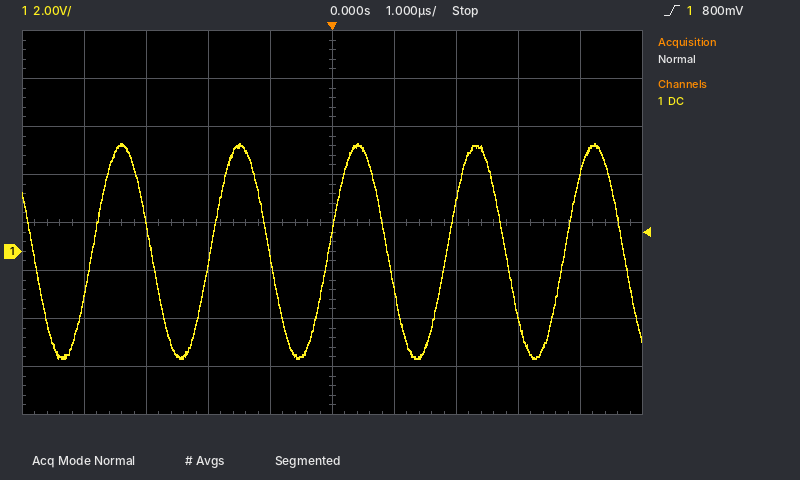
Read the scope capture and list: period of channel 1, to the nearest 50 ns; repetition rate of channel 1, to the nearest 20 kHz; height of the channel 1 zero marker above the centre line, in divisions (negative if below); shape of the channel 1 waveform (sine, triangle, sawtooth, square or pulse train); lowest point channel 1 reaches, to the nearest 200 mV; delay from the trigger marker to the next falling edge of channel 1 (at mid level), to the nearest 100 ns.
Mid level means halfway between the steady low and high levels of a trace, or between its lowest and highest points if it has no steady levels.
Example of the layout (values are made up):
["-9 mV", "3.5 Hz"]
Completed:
["1.90 µs", "520 kHz", "-0.6 div", "sine", "-4.4 V", "900 ns"]
